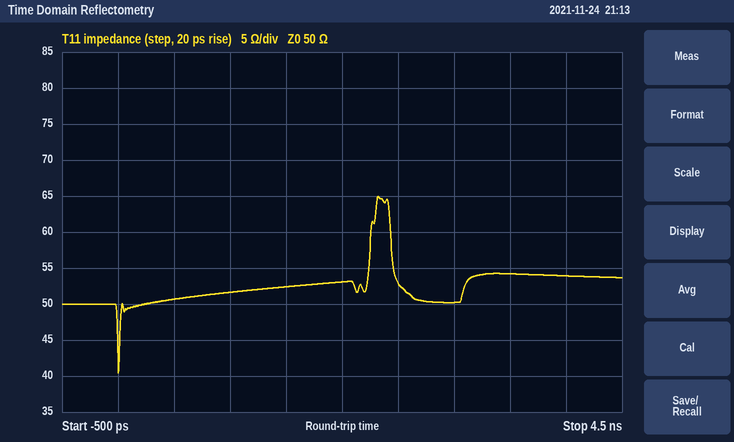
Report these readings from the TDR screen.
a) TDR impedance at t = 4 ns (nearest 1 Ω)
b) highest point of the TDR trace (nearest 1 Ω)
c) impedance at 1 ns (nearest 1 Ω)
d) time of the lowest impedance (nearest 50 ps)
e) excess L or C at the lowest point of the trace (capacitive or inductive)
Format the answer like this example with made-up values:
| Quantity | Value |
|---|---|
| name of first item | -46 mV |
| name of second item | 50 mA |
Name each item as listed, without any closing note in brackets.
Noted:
| Quantity | Value |
|---|---|
| TDR impedance at t = 4 ns | 54 Ω |
| highest point of the TDR trace | 65 Ω |
| impedance at 1 ns | 52 Ω |
| time of the lowest impedance | 0 ps |
| excess L or C at the lowest point of the trace | capacitive |
